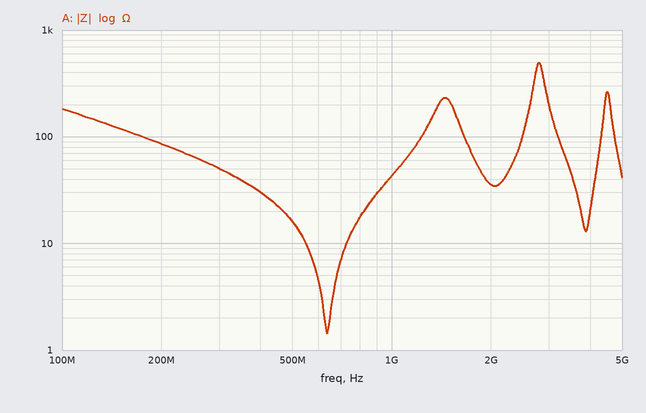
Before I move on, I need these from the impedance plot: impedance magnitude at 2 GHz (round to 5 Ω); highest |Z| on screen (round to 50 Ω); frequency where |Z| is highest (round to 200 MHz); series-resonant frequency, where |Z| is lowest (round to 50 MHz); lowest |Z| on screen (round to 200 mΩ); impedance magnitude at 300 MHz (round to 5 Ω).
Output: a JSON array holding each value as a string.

["35 Ω", "500 Ω", "2.8 GHz", "650 MHz", "1.4 Ω", "50 Ω"]
